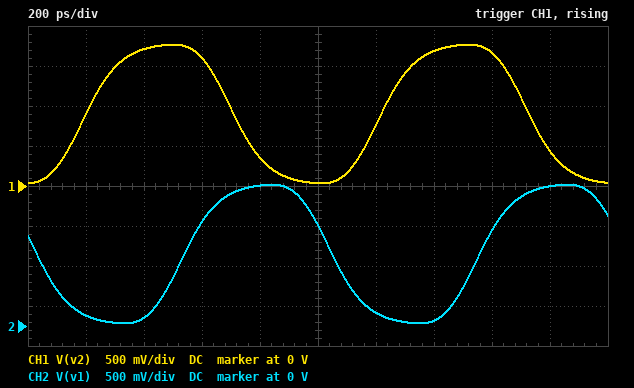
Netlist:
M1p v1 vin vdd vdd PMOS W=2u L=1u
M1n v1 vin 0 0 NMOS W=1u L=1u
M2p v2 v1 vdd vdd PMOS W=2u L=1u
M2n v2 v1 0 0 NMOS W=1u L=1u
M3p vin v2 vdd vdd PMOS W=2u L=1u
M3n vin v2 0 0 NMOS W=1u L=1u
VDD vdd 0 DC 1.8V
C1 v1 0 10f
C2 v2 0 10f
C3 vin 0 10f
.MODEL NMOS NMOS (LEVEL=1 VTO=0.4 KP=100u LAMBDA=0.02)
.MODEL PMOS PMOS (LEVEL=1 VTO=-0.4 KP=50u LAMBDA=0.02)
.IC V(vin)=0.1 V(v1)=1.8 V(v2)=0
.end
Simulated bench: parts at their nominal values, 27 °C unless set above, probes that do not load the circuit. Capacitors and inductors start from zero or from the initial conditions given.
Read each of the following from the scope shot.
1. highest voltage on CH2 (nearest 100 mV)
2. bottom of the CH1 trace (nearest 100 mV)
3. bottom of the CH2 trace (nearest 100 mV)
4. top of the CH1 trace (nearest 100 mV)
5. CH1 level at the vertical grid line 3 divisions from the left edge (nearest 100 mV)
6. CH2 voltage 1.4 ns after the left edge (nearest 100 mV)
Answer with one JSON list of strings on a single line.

["1.8 V", "0 V", "0 V", "1.8 V", "1.6 V", "100 mV"]
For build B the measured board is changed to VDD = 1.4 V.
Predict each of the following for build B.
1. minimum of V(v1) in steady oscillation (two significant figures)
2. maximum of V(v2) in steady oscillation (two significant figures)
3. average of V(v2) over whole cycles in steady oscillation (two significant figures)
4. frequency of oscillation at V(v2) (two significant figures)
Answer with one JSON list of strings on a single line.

["15 mV", "1.4 V", "700 mV", "630 MHz"]
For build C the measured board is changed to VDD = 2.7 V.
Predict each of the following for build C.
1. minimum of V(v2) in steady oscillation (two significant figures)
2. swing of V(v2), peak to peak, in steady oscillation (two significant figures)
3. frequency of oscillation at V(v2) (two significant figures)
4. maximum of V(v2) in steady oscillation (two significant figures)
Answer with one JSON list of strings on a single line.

["83 mV", "2.5 V", "1.8 GHz", "2.6 V"]
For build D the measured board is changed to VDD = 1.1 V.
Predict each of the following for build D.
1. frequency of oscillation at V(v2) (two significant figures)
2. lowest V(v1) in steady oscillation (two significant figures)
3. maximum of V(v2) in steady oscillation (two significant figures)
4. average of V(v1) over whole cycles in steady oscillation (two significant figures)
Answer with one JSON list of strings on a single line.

["390 MHz", "6.1 mV", "1.1 V", "550 mV"]
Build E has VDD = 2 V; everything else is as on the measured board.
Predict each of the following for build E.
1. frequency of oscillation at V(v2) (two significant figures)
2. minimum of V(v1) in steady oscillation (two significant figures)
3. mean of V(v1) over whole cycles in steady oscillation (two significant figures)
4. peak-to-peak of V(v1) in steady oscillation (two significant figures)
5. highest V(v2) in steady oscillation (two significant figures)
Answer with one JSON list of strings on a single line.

["1.2 GHz", "43 mV", "1.0 V", "1.9 V", "2.0 V"]
